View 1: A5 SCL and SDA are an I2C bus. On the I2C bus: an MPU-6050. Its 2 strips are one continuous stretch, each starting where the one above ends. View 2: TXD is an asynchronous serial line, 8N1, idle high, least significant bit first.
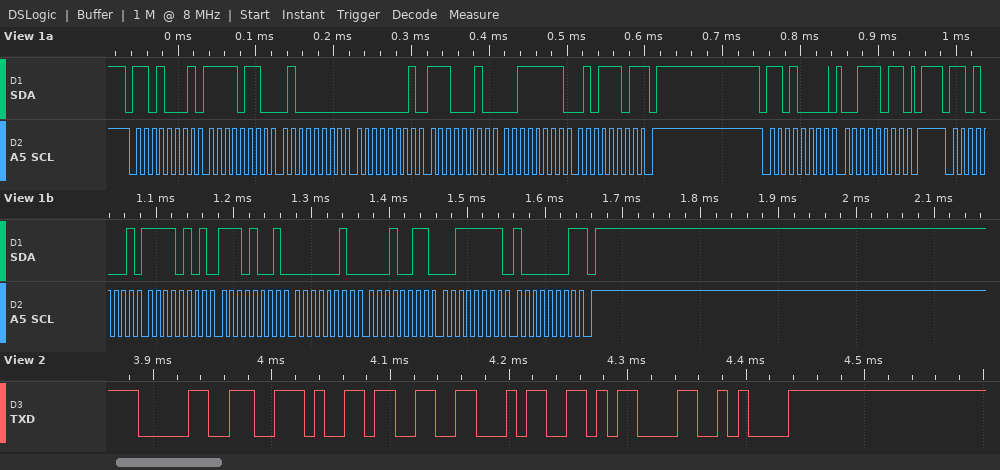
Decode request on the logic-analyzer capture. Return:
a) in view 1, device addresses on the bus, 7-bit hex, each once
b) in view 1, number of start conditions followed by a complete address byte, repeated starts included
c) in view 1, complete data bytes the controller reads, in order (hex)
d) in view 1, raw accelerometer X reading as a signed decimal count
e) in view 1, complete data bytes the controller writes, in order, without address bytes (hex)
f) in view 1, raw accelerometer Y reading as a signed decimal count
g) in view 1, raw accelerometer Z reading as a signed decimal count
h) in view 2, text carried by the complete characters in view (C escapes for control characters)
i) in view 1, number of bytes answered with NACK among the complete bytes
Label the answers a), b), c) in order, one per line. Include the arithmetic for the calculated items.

a) 0x68
b) 3
c) F6 40 01 E2 3F 5D F5 E9 02 13 3F 81
d) 0xF5E9 = -2583
e) 3B
f) 0x0213 = 531
g) 0x3F81 = 16257
h) "0.34\r\n"
i) 2
